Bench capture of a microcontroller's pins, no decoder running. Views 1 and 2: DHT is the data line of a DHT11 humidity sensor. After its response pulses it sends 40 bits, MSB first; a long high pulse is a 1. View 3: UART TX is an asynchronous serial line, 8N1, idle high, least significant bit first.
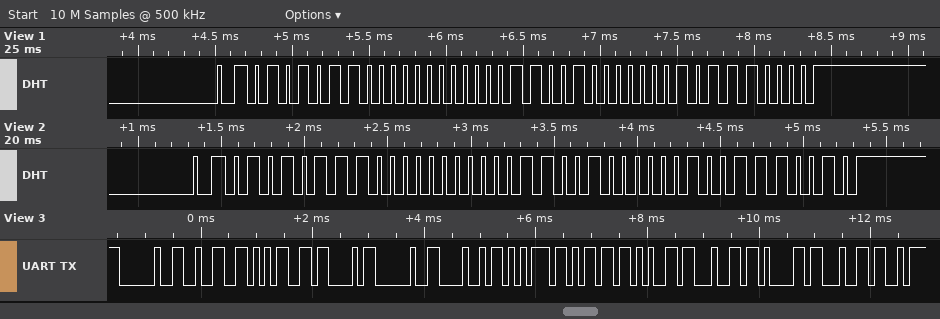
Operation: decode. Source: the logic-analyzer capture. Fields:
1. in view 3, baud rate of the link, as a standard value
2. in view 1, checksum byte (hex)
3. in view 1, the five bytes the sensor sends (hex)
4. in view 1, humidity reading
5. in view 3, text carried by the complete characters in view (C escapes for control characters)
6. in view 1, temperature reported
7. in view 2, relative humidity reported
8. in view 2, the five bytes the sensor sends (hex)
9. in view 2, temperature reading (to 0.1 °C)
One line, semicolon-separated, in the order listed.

9600 baud; 0x70; 56 00 19 01 70; 86 %; " 25C Humedad"; 25.1 °C; 87 %; 57 00 19 02 72; 25.2 °C
